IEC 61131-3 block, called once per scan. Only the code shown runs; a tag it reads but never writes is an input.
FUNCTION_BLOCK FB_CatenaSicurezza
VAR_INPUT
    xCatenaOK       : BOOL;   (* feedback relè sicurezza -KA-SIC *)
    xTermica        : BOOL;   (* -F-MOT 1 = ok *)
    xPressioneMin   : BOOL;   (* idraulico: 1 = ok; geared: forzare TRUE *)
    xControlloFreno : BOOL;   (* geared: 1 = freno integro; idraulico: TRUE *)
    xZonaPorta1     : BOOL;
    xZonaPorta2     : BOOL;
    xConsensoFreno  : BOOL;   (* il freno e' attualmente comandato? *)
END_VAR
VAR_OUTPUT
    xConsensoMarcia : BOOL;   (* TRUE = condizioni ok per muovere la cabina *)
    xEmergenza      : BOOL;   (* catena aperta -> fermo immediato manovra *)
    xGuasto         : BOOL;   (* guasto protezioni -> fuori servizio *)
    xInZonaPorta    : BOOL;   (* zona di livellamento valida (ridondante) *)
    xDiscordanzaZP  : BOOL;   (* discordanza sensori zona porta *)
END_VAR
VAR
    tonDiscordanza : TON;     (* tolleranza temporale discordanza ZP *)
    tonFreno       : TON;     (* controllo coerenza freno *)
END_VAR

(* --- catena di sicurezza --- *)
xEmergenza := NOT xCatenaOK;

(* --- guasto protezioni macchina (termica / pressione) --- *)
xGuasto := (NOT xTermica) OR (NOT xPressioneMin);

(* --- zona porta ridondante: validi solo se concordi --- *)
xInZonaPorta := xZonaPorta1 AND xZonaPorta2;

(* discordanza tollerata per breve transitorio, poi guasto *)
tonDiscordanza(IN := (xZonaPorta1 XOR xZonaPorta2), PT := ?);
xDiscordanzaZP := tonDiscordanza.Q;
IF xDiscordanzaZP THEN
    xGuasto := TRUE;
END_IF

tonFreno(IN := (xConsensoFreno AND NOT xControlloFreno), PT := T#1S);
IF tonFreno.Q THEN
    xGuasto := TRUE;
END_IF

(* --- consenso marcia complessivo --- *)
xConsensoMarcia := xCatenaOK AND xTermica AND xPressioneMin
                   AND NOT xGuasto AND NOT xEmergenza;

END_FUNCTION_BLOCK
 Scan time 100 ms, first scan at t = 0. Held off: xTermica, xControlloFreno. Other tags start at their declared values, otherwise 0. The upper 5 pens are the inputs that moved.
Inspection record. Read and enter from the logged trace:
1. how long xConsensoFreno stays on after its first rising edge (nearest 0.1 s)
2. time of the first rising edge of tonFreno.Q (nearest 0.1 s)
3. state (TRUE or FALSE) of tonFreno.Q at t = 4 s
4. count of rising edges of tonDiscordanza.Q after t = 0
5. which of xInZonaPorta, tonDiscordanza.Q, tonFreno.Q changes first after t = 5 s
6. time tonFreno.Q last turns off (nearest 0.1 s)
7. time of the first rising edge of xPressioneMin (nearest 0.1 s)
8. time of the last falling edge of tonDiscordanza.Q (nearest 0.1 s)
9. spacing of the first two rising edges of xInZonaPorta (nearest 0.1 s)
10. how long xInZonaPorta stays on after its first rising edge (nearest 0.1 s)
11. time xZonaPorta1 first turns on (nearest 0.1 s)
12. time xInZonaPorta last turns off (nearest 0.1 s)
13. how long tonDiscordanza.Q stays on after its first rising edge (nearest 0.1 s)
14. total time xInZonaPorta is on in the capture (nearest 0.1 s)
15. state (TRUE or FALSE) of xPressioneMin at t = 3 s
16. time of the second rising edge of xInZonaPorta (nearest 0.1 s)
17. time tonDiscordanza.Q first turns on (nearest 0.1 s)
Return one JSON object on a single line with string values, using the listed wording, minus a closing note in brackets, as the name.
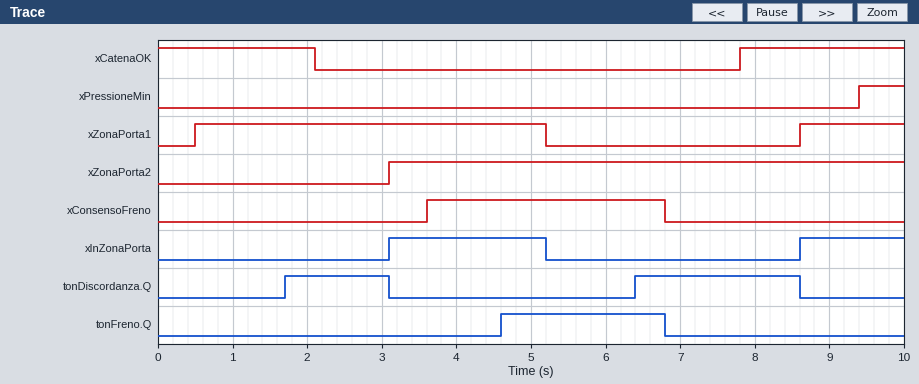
{"how long xConsensoFreno stays on after its first rising edge": "3.2 s", "time of the first rising edge of tonFreno.Q": "4.6 s", "state (TRUE or FALSE) of tonFreno.Q at t = 4 s": "FALSE", "count of rising edges of tonDiscordanza.Q after t = 0": "2", "which of xInZonaPorta, tonDiscordanza.Q, tonFreno.Q changes first after t = 5 s": "xInZonaPorta", "time tonFreno.Q last turns off": "6.8 s", "time of the first rising edge of xPressioneMin": "9.4 s", "time of the last falling edge of tonDiscordanza.Q": "8.6 s", "spacing of the first two rising edges of xInZonaPorta": "5.5 s", "how long xInZonaPorta stays on after its first rising edge": "2.1 s", "time xZonaPorta1 first turns on": "0.5 s", "time xInZonaPorta last turns off": "5.2 s", "how long tonDiscordanza.Q stays on after its first rising edge": "1.4 s", "total time xInZonaPorta is on in the capture": "3.5 s", "state (TRUE or FALSE) of xPressioneMin at t = 3 s": "FALSE", "time of the second rising edge of xInZonaPorta": "8.6 s", "time tonDiscordanza.Q first turns on": "1.7 s"}
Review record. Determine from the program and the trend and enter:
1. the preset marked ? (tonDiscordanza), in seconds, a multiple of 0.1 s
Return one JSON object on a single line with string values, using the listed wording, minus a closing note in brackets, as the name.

{"the preset marked ? (tonDiscordanza), in seconds, a multiple of 0.1 s": "1.2 s"}
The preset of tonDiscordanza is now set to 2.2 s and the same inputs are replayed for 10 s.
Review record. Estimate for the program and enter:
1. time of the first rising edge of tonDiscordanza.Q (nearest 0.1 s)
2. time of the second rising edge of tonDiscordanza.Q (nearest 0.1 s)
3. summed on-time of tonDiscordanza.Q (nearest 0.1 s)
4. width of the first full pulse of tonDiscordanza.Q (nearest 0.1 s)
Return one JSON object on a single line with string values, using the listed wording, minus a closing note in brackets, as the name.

{"time of the first rising edge of tonDiscordanza.Q": "2.7 s", "time of the second rising edge of tonDiscordanza.Q": "7.4 s", "summed on-time of tonDiscordanza.Q": "1.6 s", "width of the first full pulse of tonDiscordanza.Q": "0.4 s"}
